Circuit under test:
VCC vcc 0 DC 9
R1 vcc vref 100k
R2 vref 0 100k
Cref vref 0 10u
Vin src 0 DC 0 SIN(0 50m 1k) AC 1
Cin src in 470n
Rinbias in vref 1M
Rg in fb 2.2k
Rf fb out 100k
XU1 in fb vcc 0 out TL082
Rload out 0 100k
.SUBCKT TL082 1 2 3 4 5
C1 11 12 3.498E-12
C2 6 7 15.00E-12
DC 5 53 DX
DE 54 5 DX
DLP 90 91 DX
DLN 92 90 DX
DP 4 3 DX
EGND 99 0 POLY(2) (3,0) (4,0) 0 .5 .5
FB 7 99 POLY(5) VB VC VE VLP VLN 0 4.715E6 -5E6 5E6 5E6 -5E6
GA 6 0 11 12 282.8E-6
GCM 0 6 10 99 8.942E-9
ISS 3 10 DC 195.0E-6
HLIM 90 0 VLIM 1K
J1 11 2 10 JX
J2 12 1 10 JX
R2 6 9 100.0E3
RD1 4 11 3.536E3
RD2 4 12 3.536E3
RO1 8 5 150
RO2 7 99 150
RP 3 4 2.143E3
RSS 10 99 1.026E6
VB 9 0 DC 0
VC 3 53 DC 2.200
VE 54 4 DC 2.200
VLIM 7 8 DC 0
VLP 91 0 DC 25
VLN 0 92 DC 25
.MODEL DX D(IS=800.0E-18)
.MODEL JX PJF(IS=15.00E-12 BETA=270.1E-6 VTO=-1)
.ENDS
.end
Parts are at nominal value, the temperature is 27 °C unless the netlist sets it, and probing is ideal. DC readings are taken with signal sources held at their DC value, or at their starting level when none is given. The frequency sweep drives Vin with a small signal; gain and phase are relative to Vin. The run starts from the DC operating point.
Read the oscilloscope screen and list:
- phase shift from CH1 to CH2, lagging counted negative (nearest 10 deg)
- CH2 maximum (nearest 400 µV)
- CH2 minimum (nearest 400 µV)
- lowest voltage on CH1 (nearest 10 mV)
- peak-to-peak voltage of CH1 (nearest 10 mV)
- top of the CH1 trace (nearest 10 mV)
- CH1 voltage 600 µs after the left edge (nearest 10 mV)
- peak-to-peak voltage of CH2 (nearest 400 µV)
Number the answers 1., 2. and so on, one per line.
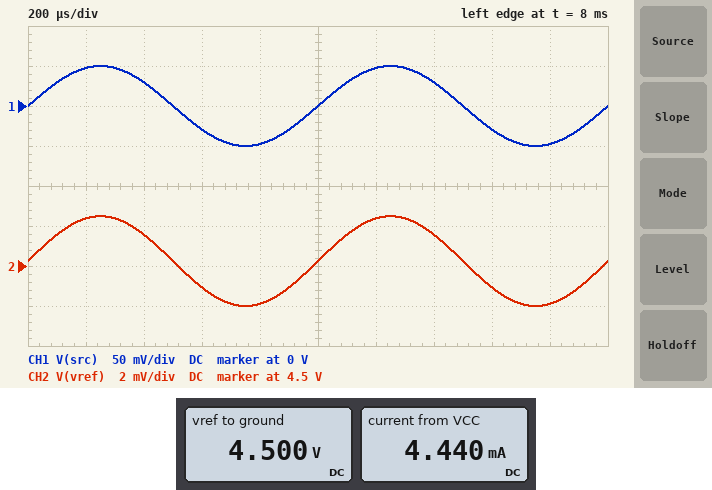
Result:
1. 0 deg
2. 4.5024 V
3. 4.4980 V
4. -50 mV
5. 100 mV
6. 50 mV
7. -30 mV
8. 4.4 mV
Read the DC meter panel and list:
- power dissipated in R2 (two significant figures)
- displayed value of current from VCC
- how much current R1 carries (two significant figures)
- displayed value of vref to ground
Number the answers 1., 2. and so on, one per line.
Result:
1. 200 µW
2. 4.440 mA
3. 45 µA
4. 4.500 V
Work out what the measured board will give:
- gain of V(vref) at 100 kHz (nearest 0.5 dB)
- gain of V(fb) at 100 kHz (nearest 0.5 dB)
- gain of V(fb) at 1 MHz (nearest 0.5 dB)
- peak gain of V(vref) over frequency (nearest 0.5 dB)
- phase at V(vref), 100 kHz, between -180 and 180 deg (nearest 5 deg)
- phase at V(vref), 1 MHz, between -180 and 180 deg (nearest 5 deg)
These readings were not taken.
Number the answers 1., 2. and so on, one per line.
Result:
1. -27.0 dB
2. -27.0 dB
3. -27.0 dB
4. -27.0 dB
5. 0 deg
6. 0 deg
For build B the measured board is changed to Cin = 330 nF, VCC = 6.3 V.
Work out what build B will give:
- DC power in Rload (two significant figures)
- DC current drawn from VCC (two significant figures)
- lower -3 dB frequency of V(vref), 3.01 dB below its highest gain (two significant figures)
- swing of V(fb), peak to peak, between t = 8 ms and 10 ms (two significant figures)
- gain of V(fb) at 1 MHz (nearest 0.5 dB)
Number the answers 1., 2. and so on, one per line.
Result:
1. 99 µW
2. 3.2 mA
3. 310 mHz
4. 3.2 mV
5. -30.0 dB
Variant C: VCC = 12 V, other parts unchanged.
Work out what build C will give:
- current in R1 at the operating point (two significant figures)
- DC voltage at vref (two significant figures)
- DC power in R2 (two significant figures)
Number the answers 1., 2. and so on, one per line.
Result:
1. 60 µA
2. 6.0 V
3. 360 µW
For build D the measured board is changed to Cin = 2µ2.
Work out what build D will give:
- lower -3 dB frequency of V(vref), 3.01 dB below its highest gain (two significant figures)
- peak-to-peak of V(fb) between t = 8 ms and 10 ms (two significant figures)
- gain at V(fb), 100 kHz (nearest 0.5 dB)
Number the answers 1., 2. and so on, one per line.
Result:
1. 260 mHz
2. 18 mV
3. -15.0 dB
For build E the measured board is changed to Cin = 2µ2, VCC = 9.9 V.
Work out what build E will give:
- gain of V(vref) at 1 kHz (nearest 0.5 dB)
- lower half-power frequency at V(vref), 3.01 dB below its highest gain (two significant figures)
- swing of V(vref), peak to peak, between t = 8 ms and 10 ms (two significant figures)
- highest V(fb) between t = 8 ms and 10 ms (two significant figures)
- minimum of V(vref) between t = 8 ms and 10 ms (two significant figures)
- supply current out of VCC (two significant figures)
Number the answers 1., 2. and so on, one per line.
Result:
1. -15.0 dB
2. 260 mHz
3. 18 mV
4. 5.0 V
5. 4.9 V
6. 4.9 mA
